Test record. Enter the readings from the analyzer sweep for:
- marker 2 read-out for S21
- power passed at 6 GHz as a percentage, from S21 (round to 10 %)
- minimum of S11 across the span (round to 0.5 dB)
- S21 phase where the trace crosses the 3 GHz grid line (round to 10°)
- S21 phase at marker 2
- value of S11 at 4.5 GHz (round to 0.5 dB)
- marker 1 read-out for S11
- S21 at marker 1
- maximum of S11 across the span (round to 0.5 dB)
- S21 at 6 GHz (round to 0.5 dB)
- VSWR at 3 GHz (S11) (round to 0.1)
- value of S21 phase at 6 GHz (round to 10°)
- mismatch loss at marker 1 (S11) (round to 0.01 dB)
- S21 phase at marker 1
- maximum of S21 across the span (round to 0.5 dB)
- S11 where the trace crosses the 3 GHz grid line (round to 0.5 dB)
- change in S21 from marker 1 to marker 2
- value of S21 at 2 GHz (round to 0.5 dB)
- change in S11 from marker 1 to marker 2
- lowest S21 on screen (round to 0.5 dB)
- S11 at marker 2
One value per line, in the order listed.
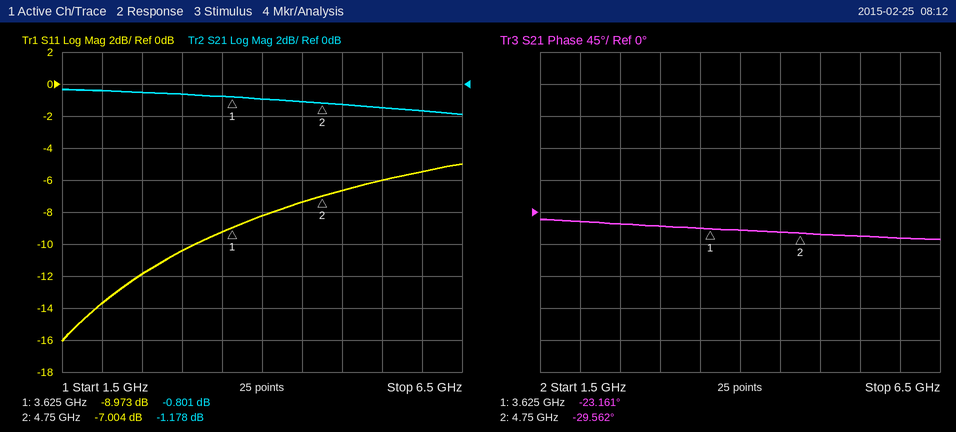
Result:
-1.178 dB
70 %
-16.0 dB
-20°
-29.562°
-7.5 dB
-8.973 dB
-0.801 dB
-5.0 dB
-1.5 dB
1.9
-40°
0.59 dB
-23.161°
-0.5 dB
-10.5 dB
-0.377 dB
-0.5 dB
1.969 dB
-2.0 dB
-7.004 dB
